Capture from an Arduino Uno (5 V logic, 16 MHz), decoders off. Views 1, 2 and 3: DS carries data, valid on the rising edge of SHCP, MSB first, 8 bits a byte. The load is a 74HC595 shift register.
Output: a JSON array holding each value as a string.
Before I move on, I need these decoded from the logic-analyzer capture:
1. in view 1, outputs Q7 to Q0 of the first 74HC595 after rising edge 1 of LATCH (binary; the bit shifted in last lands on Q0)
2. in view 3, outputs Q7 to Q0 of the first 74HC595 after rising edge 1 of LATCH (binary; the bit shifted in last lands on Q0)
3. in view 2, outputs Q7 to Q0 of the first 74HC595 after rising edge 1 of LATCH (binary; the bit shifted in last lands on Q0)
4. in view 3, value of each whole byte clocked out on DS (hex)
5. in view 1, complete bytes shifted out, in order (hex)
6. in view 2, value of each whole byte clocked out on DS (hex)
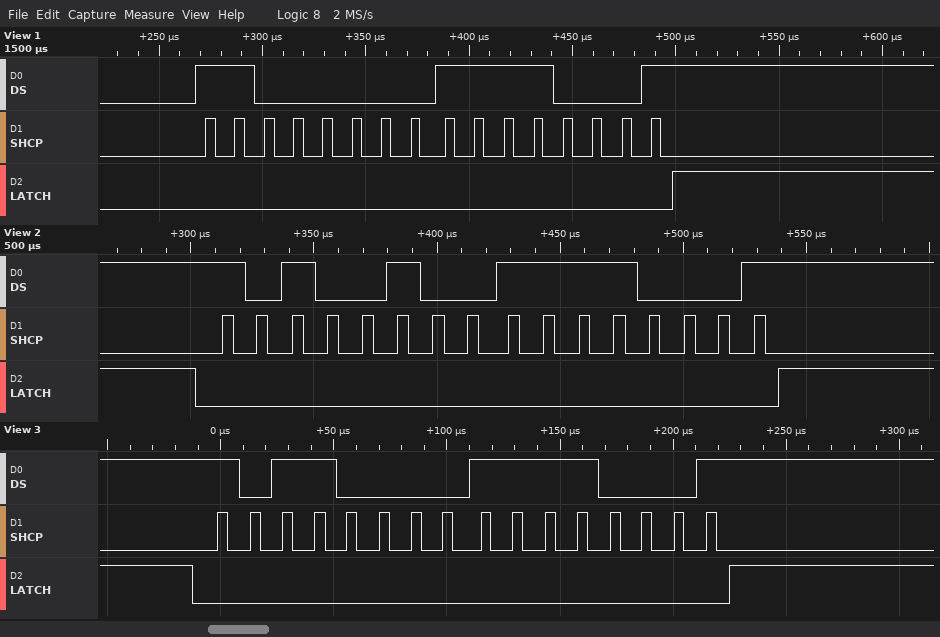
["11110001", "11110001", "11110001", "0xB0 0xF1", "0xC0 0xF1", "A4 F1"]
